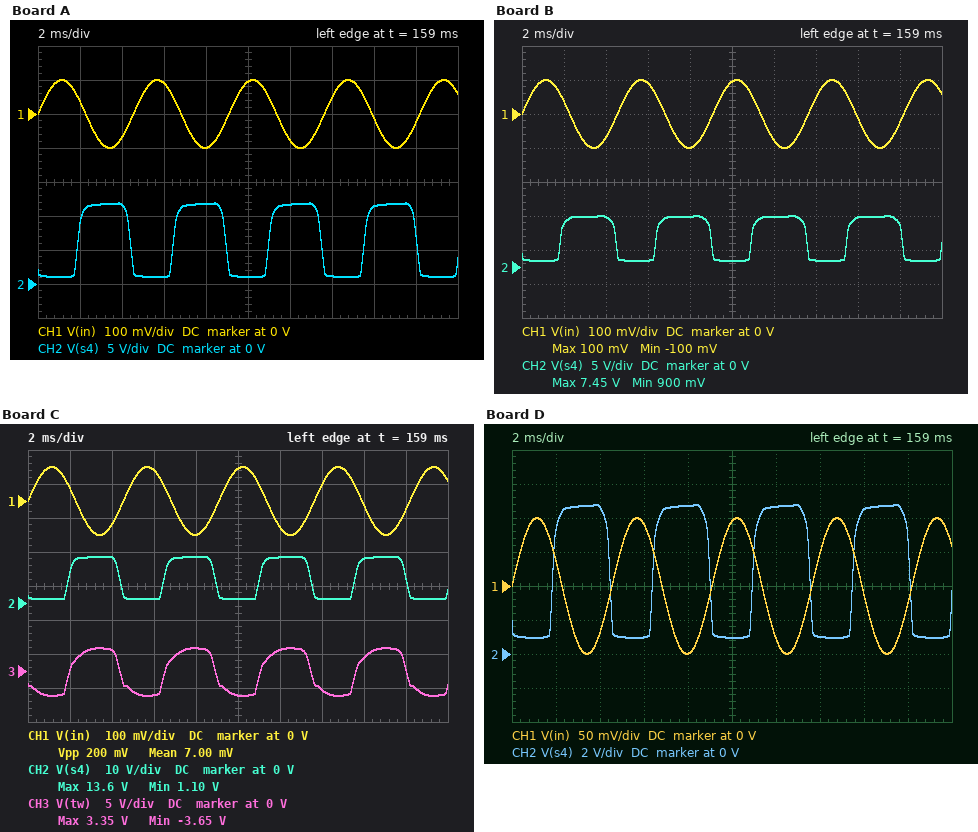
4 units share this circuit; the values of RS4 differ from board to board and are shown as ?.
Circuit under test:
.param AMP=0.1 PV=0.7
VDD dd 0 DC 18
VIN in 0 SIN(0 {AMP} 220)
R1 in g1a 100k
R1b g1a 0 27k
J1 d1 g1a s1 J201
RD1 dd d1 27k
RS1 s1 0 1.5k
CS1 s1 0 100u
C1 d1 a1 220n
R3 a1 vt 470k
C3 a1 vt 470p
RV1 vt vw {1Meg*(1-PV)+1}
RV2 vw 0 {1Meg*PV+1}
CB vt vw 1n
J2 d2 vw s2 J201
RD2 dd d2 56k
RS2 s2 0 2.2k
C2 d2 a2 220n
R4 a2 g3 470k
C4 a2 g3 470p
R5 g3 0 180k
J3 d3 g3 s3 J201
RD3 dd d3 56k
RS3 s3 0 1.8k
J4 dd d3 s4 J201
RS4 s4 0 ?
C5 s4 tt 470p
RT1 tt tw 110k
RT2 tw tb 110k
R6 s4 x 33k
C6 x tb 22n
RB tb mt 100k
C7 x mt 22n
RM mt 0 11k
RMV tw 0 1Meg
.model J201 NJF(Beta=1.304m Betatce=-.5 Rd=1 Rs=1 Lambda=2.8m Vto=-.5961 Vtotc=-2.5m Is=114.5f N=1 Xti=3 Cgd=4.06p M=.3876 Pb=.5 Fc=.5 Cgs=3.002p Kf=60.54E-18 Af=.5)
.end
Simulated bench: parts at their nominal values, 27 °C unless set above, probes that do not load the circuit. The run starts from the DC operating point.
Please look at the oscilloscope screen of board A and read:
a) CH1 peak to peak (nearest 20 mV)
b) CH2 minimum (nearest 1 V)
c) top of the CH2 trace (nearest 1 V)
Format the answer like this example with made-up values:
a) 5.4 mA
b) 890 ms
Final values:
a) 200 mV
b) 1 V
c) 12 V
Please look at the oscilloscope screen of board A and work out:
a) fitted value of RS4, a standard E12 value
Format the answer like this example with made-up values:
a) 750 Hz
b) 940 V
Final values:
a) 6.8 kΩ
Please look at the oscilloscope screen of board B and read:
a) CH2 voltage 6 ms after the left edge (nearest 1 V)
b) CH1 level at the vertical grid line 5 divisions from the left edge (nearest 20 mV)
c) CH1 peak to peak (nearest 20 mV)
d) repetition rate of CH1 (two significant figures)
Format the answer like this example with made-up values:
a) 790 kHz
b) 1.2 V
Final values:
a) 1 V
b) 100 mV
c) 200 mV
d) 220 Hz
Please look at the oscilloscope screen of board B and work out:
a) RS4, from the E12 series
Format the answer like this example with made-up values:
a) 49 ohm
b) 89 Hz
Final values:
a) 3.9 kΩ
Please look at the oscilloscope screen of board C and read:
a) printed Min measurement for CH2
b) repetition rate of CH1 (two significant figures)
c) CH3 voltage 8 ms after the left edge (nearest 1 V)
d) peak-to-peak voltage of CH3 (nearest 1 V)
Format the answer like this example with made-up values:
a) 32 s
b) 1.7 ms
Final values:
a) 1.10 V
b) 220 Hz
c) 3 V
d) 7 V
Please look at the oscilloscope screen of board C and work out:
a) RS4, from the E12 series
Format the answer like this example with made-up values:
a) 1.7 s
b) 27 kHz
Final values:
a) 8.2 kΩ
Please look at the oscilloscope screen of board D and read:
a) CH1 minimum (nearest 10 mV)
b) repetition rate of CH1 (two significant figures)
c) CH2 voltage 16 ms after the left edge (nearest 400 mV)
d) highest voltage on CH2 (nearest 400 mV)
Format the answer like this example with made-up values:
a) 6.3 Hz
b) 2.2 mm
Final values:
a) -100 mV
b) 220 Hz
c) 8.4 V
d) 8.8 V
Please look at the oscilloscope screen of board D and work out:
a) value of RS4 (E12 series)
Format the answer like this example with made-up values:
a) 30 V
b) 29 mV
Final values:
a) 4.7 kΩ
